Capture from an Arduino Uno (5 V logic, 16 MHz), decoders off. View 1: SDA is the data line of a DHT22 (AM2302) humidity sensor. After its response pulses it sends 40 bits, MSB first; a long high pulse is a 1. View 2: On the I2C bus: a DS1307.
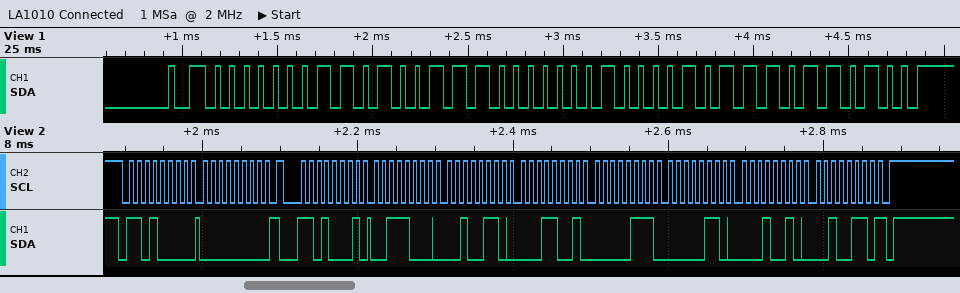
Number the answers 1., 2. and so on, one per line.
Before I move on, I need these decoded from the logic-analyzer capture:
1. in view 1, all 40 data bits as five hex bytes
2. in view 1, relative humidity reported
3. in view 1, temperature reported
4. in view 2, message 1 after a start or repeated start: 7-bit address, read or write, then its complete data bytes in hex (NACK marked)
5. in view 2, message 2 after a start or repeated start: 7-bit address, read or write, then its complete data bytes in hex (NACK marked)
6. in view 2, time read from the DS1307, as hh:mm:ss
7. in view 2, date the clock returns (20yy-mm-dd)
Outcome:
1. 01 A7 01 0B B4
2. 42.3 %
3. 26.7 °C
4. 0x68 write: 00
5. 0x68 read: 38 26 19 07 06 12 26 NACK
6. 19:26:38
7. 2026-12-06
